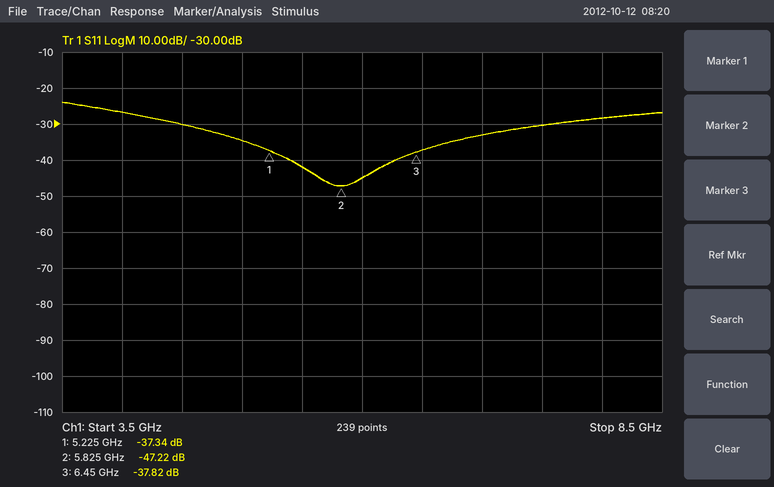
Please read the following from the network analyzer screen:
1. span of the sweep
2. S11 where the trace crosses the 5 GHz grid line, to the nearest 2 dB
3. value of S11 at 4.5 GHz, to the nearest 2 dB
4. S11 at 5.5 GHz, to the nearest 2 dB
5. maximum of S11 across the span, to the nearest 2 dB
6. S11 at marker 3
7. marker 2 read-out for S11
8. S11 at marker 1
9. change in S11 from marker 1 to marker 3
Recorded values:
5 GHz
-34 dB
-30 dB
-42 dB
-24 dB
-37.82 dB
-47.22 dB
-37.34 dB
-0.48 dB
